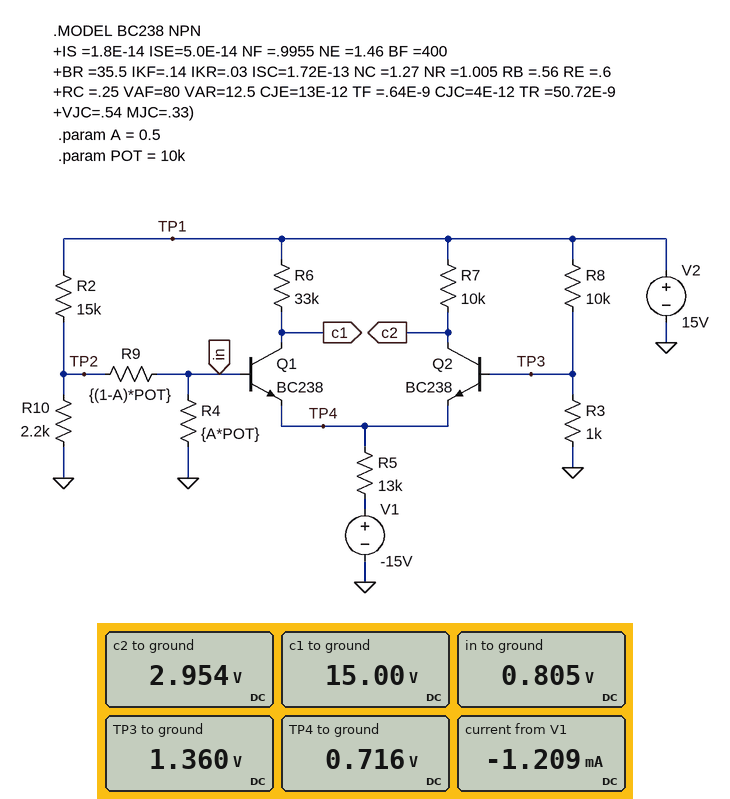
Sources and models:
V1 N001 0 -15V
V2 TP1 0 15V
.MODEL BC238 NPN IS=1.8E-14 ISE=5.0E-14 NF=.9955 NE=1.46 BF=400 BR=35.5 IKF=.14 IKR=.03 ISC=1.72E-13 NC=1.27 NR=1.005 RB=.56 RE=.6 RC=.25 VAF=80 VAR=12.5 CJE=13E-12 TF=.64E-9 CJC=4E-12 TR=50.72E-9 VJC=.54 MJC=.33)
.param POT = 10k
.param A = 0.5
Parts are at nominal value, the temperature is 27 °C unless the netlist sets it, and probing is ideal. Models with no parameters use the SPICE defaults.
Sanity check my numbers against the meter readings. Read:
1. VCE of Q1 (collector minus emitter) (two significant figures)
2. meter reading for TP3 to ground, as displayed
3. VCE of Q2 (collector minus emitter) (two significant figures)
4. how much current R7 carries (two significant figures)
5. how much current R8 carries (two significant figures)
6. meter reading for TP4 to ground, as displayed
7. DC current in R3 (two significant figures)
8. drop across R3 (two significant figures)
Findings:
14 V
1.360 V
2.2 V
1.2 mA
1.4 mA
0.716 V
1.4 mA
1.4 V
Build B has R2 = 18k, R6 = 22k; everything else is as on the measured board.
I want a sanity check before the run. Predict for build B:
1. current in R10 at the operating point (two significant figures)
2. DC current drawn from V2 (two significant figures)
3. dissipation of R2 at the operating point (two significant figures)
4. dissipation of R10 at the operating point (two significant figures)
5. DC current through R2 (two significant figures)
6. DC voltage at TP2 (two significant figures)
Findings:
620 µA
3.3 mA
10 mW
850 µW
760 µA
1.4 V
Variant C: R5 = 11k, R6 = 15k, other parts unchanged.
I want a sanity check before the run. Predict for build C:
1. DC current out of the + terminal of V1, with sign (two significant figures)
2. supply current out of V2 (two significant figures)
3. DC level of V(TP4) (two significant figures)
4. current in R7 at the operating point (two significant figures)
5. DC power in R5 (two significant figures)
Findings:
-1.4 mA
3.7 mA
710 mV
1.4 mA
22 mW
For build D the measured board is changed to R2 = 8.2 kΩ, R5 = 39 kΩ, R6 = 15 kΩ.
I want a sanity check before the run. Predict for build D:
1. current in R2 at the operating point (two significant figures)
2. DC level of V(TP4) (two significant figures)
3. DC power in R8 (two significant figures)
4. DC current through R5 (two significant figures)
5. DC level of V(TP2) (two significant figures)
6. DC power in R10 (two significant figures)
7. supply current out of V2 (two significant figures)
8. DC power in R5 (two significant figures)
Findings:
1.5 mA
760 mV
19 mW
400 µA
2.7 V
3.3 mW
3.3 mA
6.4 mW
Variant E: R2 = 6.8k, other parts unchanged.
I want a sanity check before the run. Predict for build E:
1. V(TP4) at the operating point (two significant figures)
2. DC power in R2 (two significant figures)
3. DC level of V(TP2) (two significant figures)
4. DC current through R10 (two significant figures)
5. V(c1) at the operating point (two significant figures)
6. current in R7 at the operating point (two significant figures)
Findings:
730 mV
21 mW
3.1 V
1.4 mA
740 mV
710 µA
